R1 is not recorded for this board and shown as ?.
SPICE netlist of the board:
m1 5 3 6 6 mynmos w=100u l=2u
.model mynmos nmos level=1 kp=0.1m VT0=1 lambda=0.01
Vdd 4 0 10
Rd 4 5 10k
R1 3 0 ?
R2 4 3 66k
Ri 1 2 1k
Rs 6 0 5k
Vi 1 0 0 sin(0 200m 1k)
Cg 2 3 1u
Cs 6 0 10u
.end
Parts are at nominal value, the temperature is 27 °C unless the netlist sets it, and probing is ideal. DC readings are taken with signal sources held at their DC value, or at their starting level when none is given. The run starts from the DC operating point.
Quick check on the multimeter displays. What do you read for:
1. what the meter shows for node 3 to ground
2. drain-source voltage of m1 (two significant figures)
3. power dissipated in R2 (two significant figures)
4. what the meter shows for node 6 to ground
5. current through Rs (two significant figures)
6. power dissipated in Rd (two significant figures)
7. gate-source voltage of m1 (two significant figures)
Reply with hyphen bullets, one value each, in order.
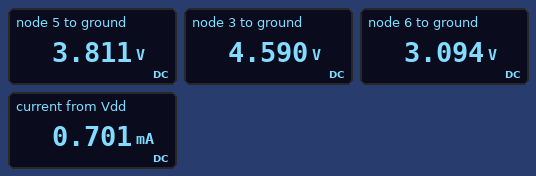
- 4.590 V
- 720 mV
- 440 µW
- 3.094 V
- 620 µA
- 3.8 mW
- 1.5 V
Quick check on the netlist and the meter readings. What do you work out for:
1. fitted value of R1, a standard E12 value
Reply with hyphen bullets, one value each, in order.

- 56 kΩ
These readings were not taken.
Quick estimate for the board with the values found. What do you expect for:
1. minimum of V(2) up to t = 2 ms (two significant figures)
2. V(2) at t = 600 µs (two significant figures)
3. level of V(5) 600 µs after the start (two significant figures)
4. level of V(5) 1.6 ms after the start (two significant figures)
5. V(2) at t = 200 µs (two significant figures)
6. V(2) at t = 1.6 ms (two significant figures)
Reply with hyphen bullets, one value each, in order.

- -190 mV
- -110 mV
- 6.3 V
- 6.1 V
- 180 mV
- -110 mV
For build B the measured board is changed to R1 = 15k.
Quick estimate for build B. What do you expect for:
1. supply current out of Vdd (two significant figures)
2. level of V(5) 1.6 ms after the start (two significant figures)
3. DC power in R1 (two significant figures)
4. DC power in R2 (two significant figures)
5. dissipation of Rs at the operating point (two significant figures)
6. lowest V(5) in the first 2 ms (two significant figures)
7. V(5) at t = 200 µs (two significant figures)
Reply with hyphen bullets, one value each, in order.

- 250 µA
- 9.8 V
- 230 µW
- 1.0 mW
- 81 µW
- 5.9 V
- 6.0 V
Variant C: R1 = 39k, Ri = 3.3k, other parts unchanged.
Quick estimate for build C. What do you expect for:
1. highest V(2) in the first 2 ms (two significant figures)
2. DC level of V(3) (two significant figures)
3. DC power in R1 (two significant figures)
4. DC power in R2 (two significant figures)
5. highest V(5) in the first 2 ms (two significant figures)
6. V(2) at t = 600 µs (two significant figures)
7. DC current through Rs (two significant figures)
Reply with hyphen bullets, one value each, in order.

- 180 mV
- 3.7 V
- 350 µW
- 600 µW
- 8.5 V
- -100 mV
- 460 µA
